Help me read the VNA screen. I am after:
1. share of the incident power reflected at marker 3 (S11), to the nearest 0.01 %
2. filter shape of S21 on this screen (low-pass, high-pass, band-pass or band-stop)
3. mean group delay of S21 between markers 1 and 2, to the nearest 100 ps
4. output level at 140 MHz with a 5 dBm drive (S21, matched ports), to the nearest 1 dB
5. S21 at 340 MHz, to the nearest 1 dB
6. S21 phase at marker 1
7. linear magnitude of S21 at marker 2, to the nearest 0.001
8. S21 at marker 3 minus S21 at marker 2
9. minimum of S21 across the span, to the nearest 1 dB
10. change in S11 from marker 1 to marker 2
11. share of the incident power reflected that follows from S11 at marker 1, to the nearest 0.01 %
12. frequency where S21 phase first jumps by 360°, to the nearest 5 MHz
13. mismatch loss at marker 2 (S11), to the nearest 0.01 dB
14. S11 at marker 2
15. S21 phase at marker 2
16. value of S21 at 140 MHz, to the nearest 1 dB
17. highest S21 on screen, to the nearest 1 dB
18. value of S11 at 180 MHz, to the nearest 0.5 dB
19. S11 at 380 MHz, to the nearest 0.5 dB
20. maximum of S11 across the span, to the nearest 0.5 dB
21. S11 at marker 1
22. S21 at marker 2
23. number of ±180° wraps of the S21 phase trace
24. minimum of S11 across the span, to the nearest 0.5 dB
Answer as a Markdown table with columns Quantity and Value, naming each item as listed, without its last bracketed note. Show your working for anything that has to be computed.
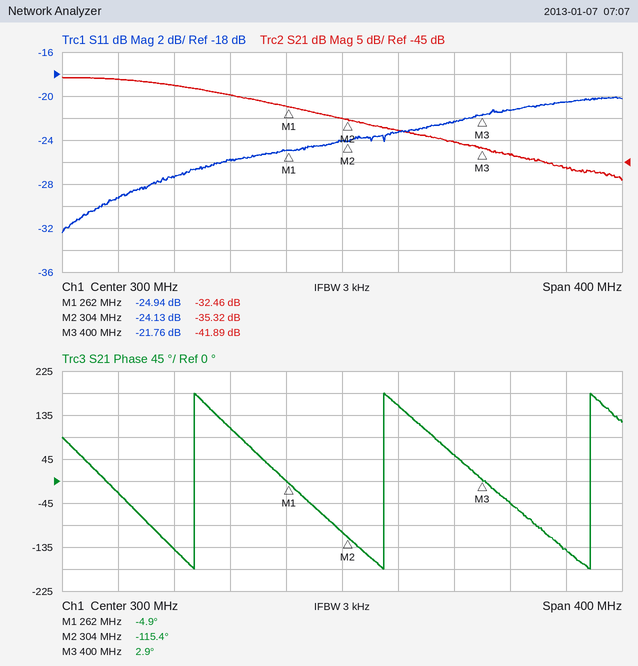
| Quantity | Value |
|---|---|
| share of the incident power reflected at marker 3 (S11), to the nearest 0.01 % | 10^(-21.76/10) ≈ 0.67 % |
| filter shape of S21 on this screen | low-pass |
| mean group delay of S21 between markers 1 and 2, to the nearest 100 ps | −(-115.4° − (-4.9°))/(360° × 42 MHz) ≈ 7.3 ns |
| output level at 140 MHz with a 5 dBm drive (S21, matched ports), to the nearest 1 dB | 5 dBm + (-26 dB) = -21 dBm |
| S21 at 340 MHz, to the nearest 1 dB | -38 dB |
| S21 phase at marker 1 | -4.9° |
| linear magnitude of S21 at marker 2, to the nearest 0.001 | 10^(-35.32/20) ≈ 0.017 |
| S21 at marker 3 minus S21 at marker 2 | -41.89 − (-35.32) = -6.57 dB |
| minimum of S21 across the span, to the nearest 1 dB | -49 dB |
| change in S11 from marker 1 to marker 2 | -24.13 − (-24.94) = 0.81 dB |
| share of the incident power reflected that follows from S11 at marker 1, to the nearest 0.01 % | 10^(-24.94/10) ≈ 0.32 % |
| frequency where S21 phase first jumps by 360°, to the nearest 5 MHz | 195 MHz |
| mismatch loss at marker 2 (S11), to the nearest 0.01 dB | −10 log10(1 − 10^(-24.13/10)) ≈ 0.02 dB |
| S11 at marker 2 | -24.13 dB |
| S21 phase at marker 2 | -115.4° |
| value of S21 at 140 MHz, to the nearest 1 dB | -26 dB |
| highest S21 on screen, to the nearest 1 dB | -26 dB |
| value of S11 at 180 MHz, to the nearest 0.5 dB | -27.5 dB |
| S11 at 380 MHz, to the nearest 0.5 dB | -22.5 dB |
| maximum of S11 across the span, to the nearest 0.5 dB | -20.0 dB |
| S11 at marker 1 | -24.94 dB |
| S21 at marker 2 | -35.32 dB |
| number of ±180° wraps of the S21 phase trace | 3 |
| minimum of S11 across the span, to the nearest 0.5 dB | -32.5 dB |
